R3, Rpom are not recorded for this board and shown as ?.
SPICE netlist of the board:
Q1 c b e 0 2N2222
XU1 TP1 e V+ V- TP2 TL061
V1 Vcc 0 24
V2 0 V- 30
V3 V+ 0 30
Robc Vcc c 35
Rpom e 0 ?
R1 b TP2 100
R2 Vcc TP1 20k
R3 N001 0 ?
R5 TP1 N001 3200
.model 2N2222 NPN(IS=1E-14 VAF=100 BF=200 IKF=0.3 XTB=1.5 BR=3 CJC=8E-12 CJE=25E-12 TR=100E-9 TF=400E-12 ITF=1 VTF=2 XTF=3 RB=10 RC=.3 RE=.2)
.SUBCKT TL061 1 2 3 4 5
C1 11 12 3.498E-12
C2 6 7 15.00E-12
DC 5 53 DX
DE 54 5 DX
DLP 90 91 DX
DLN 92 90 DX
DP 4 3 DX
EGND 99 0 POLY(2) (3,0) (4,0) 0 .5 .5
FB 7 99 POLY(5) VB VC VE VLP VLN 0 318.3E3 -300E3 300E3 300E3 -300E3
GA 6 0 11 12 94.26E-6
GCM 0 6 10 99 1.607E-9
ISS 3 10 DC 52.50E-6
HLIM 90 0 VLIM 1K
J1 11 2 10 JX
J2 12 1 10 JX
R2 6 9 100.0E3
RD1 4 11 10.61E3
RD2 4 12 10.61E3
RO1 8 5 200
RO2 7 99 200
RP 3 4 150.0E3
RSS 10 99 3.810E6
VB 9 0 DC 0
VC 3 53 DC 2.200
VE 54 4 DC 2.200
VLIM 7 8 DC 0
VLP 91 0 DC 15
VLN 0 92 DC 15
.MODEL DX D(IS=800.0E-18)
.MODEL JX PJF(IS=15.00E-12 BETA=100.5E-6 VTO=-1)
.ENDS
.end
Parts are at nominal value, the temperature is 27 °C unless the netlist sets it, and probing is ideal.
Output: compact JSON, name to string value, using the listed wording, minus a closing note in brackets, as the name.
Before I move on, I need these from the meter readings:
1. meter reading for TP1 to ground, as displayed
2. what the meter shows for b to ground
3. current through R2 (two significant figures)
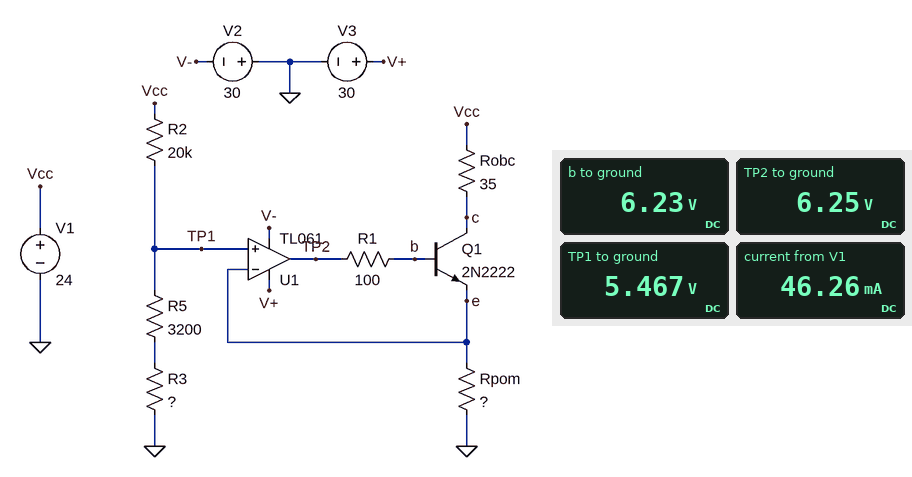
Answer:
{"meter reading for TP1 to ground, as displayed": "5.467 V", "what the meter shows for b to ground": "6.23 V", "current through R2": "930 µA"}
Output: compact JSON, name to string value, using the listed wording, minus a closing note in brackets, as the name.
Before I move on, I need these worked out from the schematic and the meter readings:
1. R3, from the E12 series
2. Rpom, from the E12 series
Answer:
{"R3, from the E12 series": "2.7 kΩ", "Rpom, from the E12 series": "120 Ω"}
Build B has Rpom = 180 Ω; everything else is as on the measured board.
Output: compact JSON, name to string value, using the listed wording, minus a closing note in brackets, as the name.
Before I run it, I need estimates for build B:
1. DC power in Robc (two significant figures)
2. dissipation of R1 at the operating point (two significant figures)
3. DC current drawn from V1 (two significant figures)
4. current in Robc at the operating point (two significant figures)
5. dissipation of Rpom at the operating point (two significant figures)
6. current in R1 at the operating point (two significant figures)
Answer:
{"DC power in Robc": "32 mW", "dissipation of R1 at the operating point": "2.0 µW", "DC current drawn from V1": "31 mA", "current in Robc at the operating point": "30 mA", "dissipation of Rpom at the operating point": "170 mW", "current in R1 at the operating point": "140 µA"}
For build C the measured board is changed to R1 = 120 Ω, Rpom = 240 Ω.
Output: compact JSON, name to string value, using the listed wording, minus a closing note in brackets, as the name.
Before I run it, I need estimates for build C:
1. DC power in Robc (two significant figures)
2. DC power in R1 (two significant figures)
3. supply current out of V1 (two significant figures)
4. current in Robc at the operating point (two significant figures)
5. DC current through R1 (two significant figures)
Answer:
{"DC power in Robc": "18 mW", "DC power in R1": "1.3 µW", "supply current out of V1": "24 mA", "current in Robc at the operating point": "23 mA", "DC current through R1": "100 µA"}
